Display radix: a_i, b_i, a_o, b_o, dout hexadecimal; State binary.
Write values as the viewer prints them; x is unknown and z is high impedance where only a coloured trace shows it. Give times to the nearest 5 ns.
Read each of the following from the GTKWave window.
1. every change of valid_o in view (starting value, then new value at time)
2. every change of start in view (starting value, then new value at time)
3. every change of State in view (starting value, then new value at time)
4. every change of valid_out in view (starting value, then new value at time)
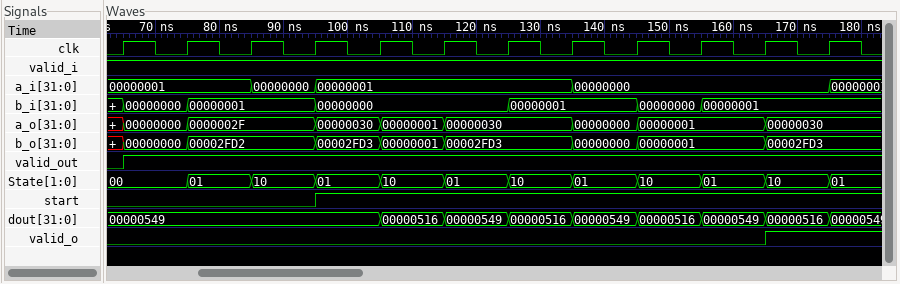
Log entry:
0, 1 at 165 ns
0, 1 at 95 ns
00, 01 at 75 ns, 10 at 85 ns, 01 at 95 ns, 10 at 105 ns, 01 at 115 ns, 10 at 125 ns, 01 at 135 ns, 10 at 145 ns, 01 at 155 ns, 10 at 165 ns, 01 at 175 ns
0, 1 at 65 ns
